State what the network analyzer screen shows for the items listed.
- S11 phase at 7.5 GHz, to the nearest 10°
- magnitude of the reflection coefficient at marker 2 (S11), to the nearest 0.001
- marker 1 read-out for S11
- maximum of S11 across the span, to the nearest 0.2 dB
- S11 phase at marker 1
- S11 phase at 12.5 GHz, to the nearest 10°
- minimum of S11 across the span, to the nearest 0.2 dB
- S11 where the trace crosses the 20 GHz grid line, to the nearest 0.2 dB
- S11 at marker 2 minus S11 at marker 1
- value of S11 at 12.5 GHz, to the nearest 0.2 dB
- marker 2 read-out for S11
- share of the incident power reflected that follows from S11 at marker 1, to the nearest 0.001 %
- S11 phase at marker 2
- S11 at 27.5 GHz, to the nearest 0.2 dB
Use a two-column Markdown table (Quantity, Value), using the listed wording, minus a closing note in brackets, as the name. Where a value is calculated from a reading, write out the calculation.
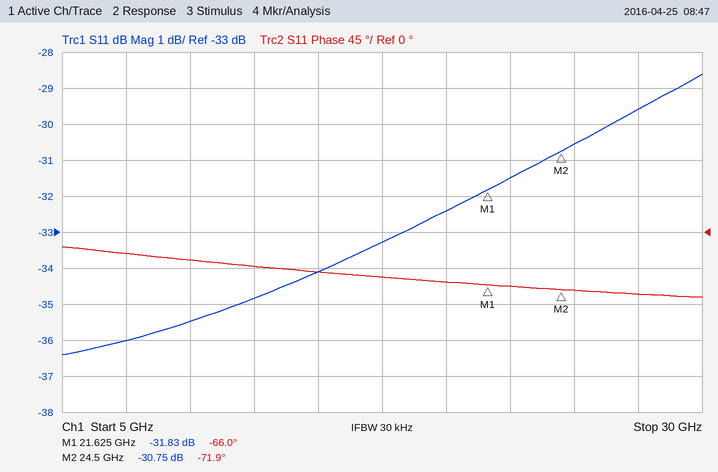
| Quantity | Value |
|---|---|
| S11 phase at 7.5 GHz, to the nearest 10° | -30° |
| magnitude of the reflection coefficient at marker 2 (S11), to the nearest 0.001 | 10^(-30.75/20) ≈ 0.029 |
| marker 1 read-out for S11 | -31.83 dB |
| maximum of S11 across the span, to the nearest 0.2 dB | -28.6 dB |
| S11 phase at marker 1 | -66.0° |
| S11 phase at 12.5 GHz, to the nearest 10° | -40° |
| minimum of S11 across the span, to the nearest 0.2 dB | -36.4 dB |
| S11 where the trace crosses the 20 GHz grid line, to the nearest 0.2 dB | -32.4 dB |
| S11 at marker 2 minus S11 at marker 1 | -30.75 − (-31.83) = 1.08 dB |
| value of S11 at 12.5 GHz, to the nearest 0.2 dB | -34.8 dB |
| marker 2 read-out for S11 | -30.75 dB |
| share of the incident power reflected that follows from S11 at marker 1, to the nearest 0.001 % | 10^(-31.83/10) ≈ 0.066 % |
| S11 phase at marker 2 | -71.9° |
| S11 at 27.5 GHz, to the nearest 0.2 dB | -29.6 dB |
